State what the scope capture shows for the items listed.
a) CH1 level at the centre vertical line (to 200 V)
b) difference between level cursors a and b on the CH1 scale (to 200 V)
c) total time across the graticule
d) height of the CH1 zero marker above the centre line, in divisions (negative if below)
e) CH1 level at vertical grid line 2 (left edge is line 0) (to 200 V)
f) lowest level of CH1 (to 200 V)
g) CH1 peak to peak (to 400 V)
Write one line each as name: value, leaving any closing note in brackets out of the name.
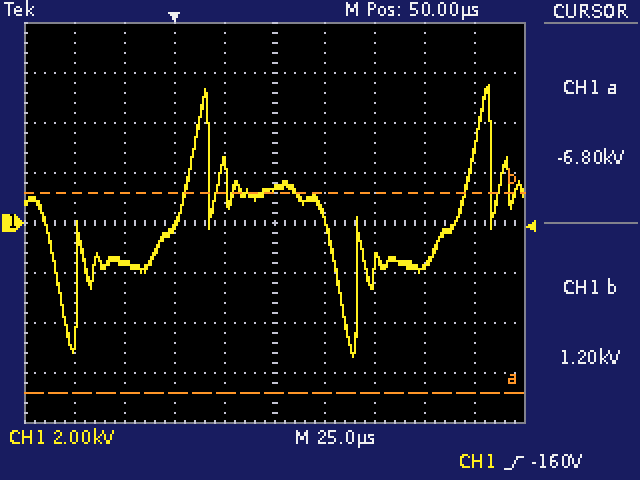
CH1 level at the centre vertical line: 1.4 kV
difference between level cursors a and b on the CH1 scale: 8.0 kV
total time across the graticule: 250 µs
height of the CH1 zero marker above the centre line, in divisions: 0.0 div
CH1 level at vertical grid line 2 (left edge is line 0): -1.6 kV
lowest level of CH1: -5.4 kV
CH1 peak to peak: 10.8 kV
